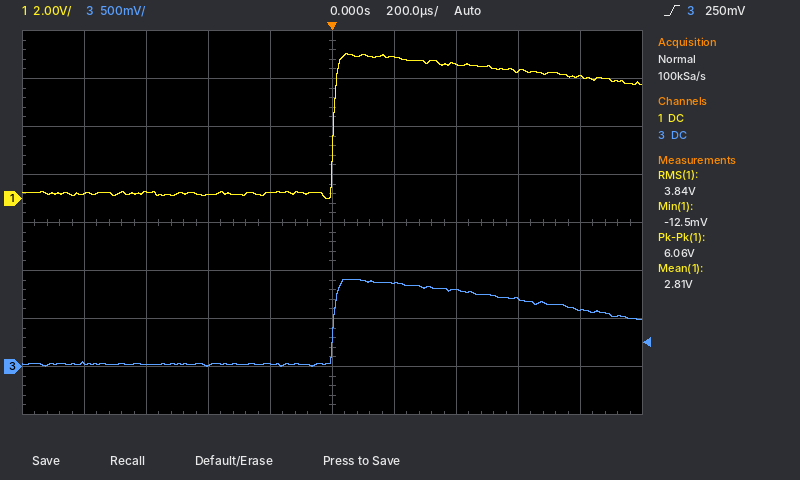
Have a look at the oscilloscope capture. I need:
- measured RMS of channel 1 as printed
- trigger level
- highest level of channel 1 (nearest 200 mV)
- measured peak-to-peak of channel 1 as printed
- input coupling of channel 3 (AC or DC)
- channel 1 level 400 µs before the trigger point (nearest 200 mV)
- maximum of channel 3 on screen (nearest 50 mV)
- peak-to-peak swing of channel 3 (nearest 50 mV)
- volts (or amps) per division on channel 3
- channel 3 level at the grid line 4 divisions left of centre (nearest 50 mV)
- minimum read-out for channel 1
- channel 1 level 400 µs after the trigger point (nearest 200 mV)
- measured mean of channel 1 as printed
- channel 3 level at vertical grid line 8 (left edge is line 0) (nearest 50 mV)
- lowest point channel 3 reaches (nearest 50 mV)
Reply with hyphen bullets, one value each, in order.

- 3.84 V
- 250 mV
- 6.0 V
- 6.06 V
- DC
- 200 mV
- 900 mV
- 900 mV
- 500 mV
- 50 mV
- -12.5 mV
- 5.6 V
- 2.81 V
- 700 mV
- 0 mV
